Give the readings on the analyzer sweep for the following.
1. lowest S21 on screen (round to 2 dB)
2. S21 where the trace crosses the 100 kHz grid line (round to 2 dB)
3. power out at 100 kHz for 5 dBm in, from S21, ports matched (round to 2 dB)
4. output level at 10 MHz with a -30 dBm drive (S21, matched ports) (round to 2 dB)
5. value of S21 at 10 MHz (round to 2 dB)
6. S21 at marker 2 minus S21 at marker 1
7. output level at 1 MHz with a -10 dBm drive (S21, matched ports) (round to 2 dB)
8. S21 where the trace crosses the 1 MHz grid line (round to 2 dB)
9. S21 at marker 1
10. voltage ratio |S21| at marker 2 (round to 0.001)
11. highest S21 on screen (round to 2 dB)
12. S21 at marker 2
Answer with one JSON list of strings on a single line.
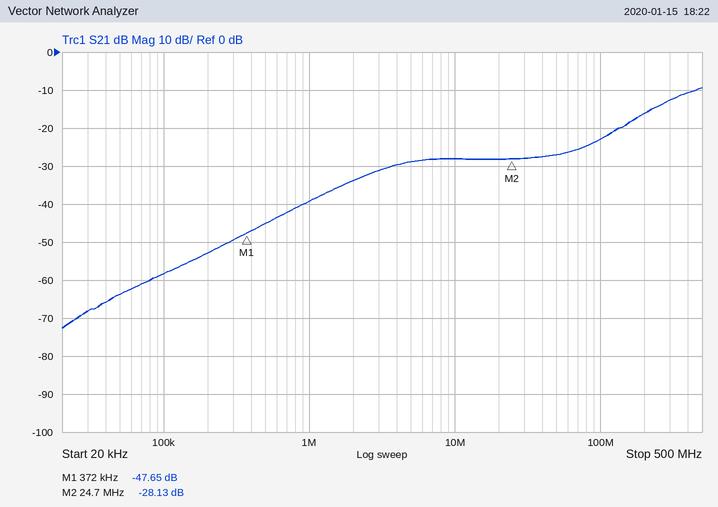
["-72 dB", "-58 dB", "-54 dBm", "-58 dBm", "-28 dB", "19.52 dB", "-50 dBm", "-40 dB", "-47.65 dB", "0.039", "-10 dB", "-28.13 dB"]
